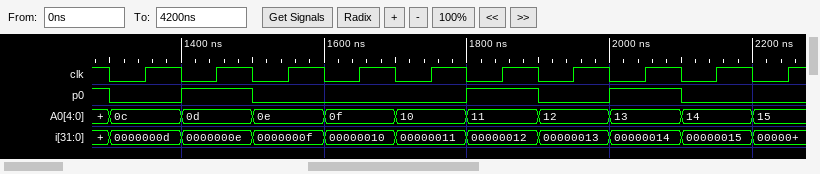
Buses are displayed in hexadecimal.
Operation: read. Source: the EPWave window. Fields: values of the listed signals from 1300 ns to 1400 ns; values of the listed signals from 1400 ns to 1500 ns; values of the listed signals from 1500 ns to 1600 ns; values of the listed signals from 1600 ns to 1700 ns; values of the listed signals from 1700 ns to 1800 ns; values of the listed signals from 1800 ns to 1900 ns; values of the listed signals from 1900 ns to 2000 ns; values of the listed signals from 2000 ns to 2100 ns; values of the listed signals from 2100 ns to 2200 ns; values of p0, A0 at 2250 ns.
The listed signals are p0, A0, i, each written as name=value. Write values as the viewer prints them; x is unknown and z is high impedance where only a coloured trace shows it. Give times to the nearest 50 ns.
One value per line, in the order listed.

p0=0, A0=0c, i=0000000d
p0=1, A0=0d, i=0000000e
p0=0, A0=0e, i=0000000f
p0=0, A0=0f, i=00000010
p0=0, A0=10, i=00000011
p0=1, A0=11, i=00000012
p0=0, A0=12, i=00000013
p0=1, A0=13, i=00000014
p0=0, A0=14, i=00000015
p0=0, A0=15
